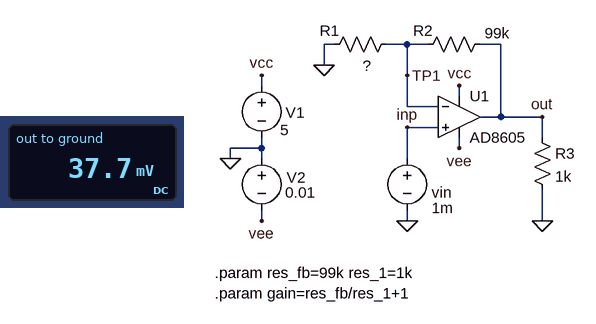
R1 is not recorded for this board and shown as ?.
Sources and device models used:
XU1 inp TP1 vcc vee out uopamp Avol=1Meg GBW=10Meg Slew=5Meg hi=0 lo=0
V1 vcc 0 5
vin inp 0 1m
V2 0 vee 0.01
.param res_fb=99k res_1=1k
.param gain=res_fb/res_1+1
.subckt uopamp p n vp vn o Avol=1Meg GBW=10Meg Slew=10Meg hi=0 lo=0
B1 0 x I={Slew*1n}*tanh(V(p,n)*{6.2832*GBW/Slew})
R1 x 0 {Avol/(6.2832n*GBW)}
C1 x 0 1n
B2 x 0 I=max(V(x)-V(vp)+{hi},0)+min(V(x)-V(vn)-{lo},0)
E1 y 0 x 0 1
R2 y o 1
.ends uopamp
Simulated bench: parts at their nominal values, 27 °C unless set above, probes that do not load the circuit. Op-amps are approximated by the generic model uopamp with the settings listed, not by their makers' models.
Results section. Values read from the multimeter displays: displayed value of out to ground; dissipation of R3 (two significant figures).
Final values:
37.7 mV
1.4 µW
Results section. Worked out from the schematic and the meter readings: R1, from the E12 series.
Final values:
2.7 kΩ
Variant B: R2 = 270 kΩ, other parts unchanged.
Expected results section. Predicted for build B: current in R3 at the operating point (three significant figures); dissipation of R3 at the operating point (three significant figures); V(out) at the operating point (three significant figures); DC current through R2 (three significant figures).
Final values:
101 µA
10.2 µW
101 mV
370 nA
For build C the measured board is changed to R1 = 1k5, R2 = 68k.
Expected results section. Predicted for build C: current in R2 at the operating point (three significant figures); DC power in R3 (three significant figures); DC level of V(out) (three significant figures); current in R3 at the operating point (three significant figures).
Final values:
667 nA
2.15 µW
46.3 mV
46.3 µA
